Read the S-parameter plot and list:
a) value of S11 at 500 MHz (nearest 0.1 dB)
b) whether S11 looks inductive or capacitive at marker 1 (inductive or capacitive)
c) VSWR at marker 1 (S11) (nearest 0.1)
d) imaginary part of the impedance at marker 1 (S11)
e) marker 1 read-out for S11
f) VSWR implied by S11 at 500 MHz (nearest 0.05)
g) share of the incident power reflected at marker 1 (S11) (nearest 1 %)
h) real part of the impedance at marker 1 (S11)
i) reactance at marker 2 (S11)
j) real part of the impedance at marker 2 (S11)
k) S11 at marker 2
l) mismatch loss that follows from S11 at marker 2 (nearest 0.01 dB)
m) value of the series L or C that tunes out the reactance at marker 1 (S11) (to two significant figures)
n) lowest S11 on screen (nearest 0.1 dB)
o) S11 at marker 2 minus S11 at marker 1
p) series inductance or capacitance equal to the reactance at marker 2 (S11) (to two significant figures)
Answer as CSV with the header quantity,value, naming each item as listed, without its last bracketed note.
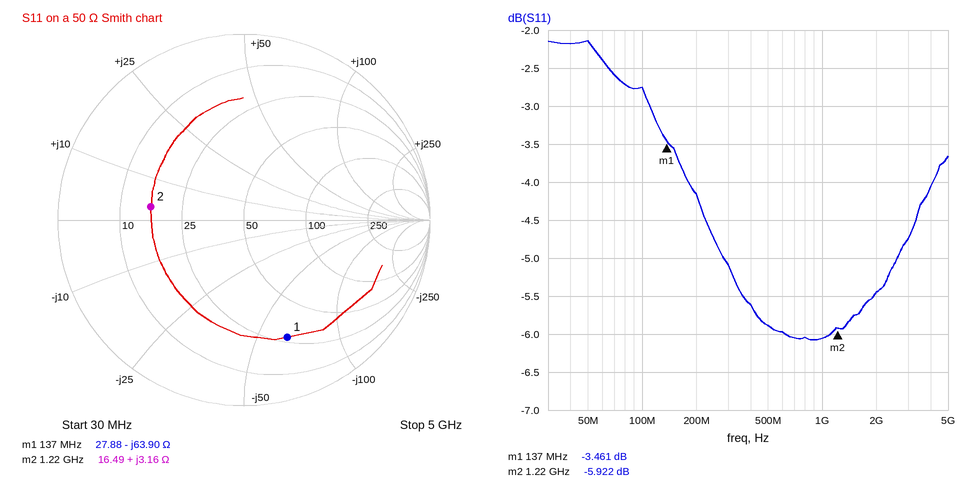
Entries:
quantity,value
value of S11 at 500 MHz,-5.9 dB
whether S11 looks inductive or capacitive at marker 1,capacitive
VSWR at marker 1 (S11),5.1
imaginary part of the impedance at marker 1,-63.90 Ω
marker 1 read-out for S11,-3.461 dB
VSWR implied by S11 at 500 MHz,3.05
share of the incident power reflected at marker 1 (S11),45 %
real part of the impedance at marker 1,27.88 Ω
reactance at marker 2,+3.16 Ω
real part of the impedance at marker 2,16.49 Ω
S11 at marker 2,-5.922 dB
mismatch loss that follows from S11 at marker 2,1.28 dB
value of the series L or C that tunes out the reactance at marker 1 (S11),74 nH
lowest S11 on screen,-6.1 dB
S11 at marker 2 minus S11 at marker 1,-2.461 dB
series inductance or capacitance equal to the reactance at marker 2 (S11),410 pH
